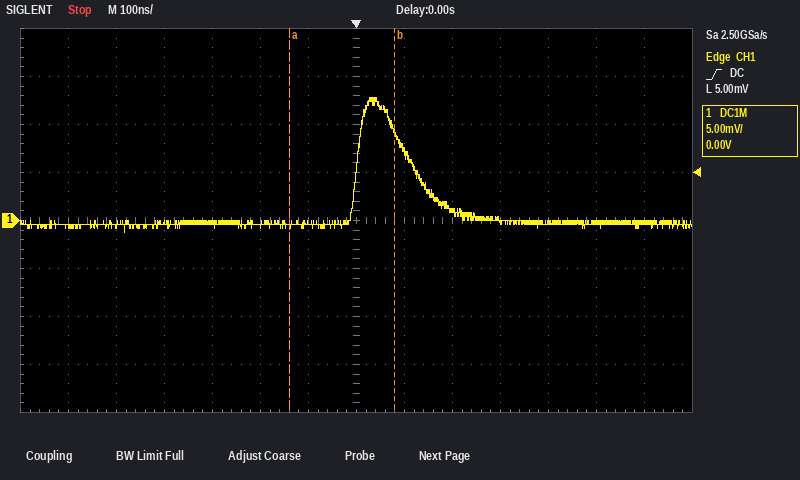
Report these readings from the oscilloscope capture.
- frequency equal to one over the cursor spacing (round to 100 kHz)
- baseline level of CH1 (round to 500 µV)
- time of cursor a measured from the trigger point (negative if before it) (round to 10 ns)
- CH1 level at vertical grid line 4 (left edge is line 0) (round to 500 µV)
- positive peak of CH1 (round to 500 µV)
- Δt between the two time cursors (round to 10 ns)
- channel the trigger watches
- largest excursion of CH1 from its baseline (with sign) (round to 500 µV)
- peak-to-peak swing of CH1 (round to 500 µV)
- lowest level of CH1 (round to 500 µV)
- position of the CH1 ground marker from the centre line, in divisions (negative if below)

4.5 MHz
0.0 mV
-140 ns
0.0 mV
13.0 mV
220 ns
CH1
+13.0 mV
14.0 mV
-1.0 mV
0.0 div
